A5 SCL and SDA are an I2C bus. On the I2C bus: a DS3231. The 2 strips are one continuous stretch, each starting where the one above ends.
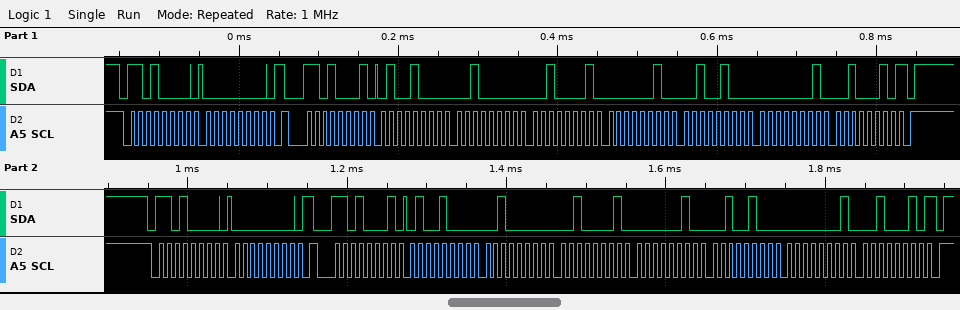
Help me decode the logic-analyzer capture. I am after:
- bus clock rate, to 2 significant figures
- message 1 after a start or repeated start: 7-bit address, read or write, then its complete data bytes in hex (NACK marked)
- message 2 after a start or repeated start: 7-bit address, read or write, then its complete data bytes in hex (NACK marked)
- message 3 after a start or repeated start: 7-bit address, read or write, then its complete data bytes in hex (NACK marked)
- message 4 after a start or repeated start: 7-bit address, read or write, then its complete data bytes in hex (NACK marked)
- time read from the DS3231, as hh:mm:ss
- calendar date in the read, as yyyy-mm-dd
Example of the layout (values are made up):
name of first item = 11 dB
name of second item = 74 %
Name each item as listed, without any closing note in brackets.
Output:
bus clock rate, to 2 significant figures = 100 kHz
message 1 after a start or repeated start: 7-bit address, read or write, then its complete data bytes in hex = 0x68 write: 00
message 2 after a start or repeated start: 7-bit address, read or write, then its complete data bytes in hex = 0x68 read: 48 20 21 02 24 01 22 NACK
message 3 after a start or repeated start: 7-bit address, read or write, then its complete data bytes in hex = 0x68 write: 00
message 4 after a start or repeated start: 7-bit address, read or write, then its complete data bytes in hex = 0x68 read: 48 20 21 02 24 01 22 NACK
time read from the DS3231, as hh:mm:ss = 21:20:48
calendar date in the read, as yyyy-mm-dd = 2022-01-24
